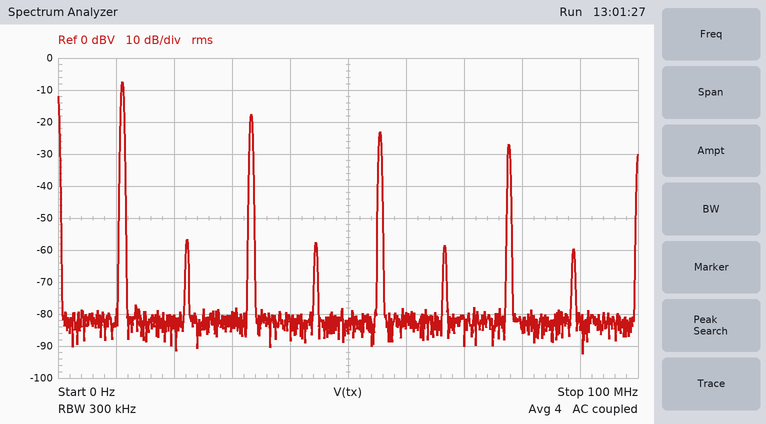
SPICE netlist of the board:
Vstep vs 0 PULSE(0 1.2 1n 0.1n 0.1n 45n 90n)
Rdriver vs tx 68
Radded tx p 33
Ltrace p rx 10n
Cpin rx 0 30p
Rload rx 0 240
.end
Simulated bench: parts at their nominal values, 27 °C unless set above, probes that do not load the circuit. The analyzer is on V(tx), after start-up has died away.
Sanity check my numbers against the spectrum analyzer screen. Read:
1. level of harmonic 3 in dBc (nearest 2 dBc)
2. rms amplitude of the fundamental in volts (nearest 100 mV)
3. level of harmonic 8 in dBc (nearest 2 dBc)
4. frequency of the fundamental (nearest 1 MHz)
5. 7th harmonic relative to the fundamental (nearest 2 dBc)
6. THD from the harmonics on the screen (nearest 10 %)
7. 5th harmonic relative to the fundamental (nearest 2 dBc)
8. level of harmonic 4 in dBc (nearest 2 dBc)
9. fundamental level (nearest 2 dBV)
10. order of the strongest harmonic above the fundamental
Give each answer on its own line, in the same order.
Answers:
-10 dBc
400 mV
-52 dBc
11 MHz
-20 dBc
40 %
-16 dBc
-50 dBc
-8 dBV
3
